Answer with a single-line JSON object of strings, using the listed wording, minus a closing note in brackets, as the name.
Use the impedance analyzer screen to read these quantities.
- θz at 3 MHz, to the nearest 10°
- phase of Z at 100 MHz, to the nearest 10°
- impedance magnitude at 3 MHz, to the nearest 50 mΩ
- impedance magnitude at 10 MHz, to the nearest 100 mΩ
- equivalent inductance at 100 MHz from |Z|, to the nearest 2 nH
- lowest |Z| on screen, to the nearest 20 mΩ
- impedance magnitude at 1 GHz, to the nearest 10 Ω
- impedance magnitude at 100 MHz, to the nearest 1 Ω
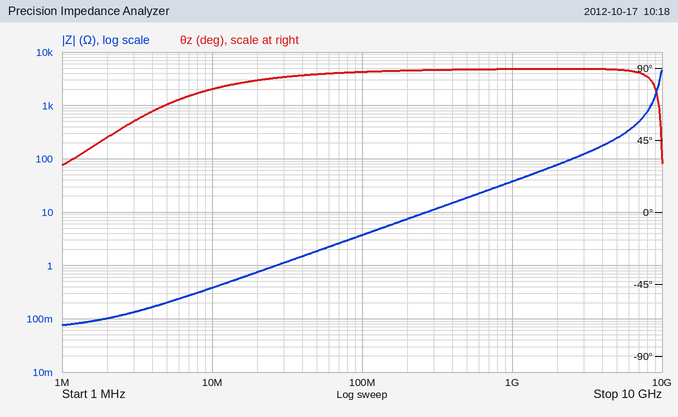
{"θz at 3 MHz, to the nearest 10°": "60°", "phase of Z at 100 MHz, to the nearest 10°": "90°", "impedance magnitude at 3 MHz, to the nearest 50 mΩ": "150 mΩ", "impedance magnitude at 10 MHz, to the nearest 100 mΩ": "400 mΩ", "equivalent inductance at 100 MHz from |Z|, to the nearest 2 nH": "6 nH", "lowest |Z| on screen, to the nearest 20 mΩ": "80 mΩ", "impedance magnitude at 1 GHz, to the nearest 10 Ω": "40 Ω", "impedance magnitude at 100 MHz, to the nearest 1 Ω": "4 Ω"}
